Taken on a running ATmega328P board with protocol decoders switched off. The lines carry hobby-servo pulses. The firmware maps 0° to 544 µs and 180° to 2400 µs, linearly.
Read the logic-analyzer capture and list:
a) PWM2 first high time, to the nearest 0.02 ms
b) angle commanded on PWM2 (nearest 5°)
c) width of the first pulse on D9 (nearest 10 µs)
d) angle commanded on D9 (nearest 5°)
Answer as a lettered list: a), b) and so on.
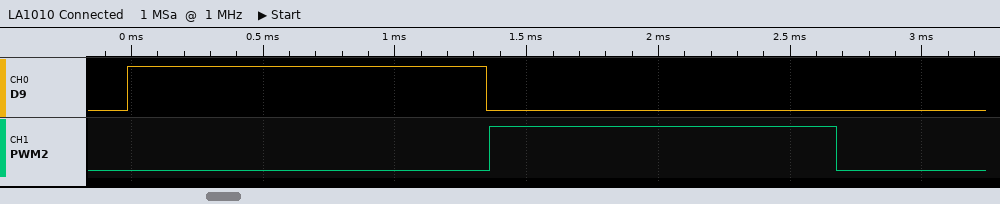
a) 1.32 ms
b) 75°
c) 1360 µs
d) 80°
